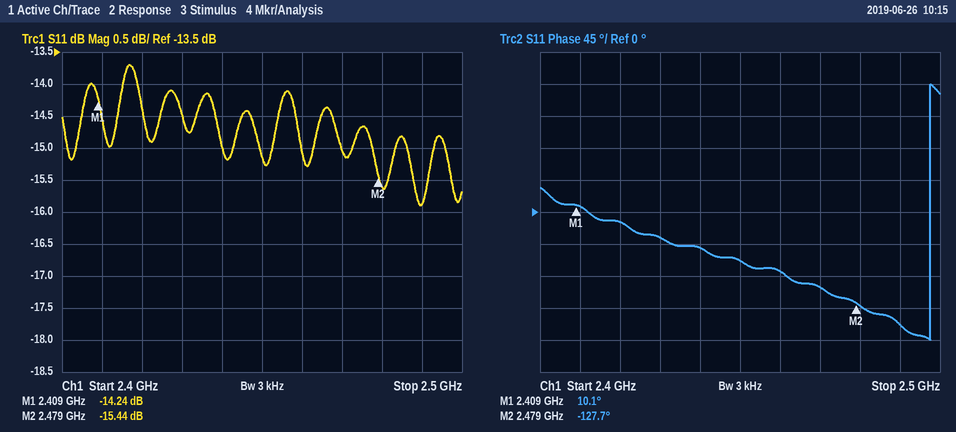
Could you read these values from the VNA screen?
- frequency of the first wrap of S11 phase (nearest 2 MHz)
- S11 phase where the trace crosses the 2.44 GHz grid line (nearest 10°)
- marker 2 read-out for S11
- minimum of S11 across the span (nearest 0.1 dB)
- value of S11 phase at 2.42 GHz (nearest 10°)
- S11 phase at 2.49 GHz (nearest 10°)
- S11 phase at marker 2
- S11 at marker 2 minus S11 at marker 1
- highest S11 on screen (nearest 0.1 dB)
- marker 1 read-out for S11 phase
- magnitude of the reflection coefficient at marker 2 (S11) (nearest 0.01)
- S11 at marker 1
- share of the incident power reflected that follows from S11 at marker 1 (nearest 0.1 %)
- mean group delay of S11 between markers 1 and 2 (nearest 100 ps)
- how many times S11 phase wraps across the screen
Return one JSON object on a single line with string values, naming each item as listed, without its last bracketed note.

{"frequency of the first wrap of S11 phase": "2.498 GHz", "S11 phase where the trace crosses the 2.44 GHz grid line": "-50°", "marker 2 read-out for S11": "-15.44 dB", "minimum of S11 across the span": "-15.9 dB", "value of S11 phase at 2.42 GHz": "-10°", "S11 phase at 2.49 GHz": "-160°", "S11 phase at marker 2": "-127.7°", "S11 at marker 2 minus S11 at marker 1": "-1.20 dB", "highest S11 on screen": "-13.7 dB", "marker 1 read-out for S11 phase": "10.1°", "magnitude of the reflection coefficient at marker 2 (S11)": "0.17", "S11 at marker 1": "-14.24 dB", "share of the incident power reflected that follows from S11 at marker 1": "3.8 %", "mean group delay of S11 between markers 1 and 2": "5.5 ns", "how many times S11 phase wraps across the screen": "1"}
